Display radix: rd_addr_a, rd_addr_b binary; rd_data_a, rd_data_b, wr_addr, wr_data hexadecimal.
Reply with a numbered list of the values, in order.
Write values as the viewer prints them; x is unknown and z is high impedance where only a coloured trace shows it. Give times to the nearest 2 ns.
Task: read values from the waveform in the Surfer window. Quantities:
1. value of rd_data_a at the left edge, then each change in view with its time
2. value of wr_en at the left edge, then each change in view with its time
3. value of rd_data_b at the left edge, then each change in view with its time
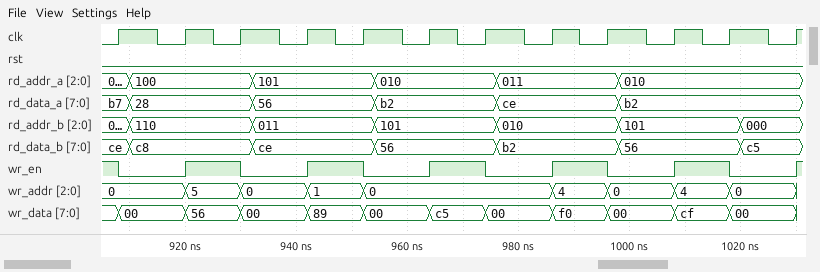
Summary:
1. b7, 28 at 910 ns, 56 at 932 ns, b2 at 954 ns, ce at 976 ns, b2 at 998 ns
2. 1, 0 at 908 ns, 1 at 920 ns, 0 at 930 ns, 1 at 942 ns, 0 at 952 ns, 1 at 964 ns, 0 at 974 ns, 1 at 986 ns, 0 at 996 ns, 1 at 1008 ns, 0 at 1018 ns, 1 at 1030 ns
3. ce, c8 at 910 ns, ce at 932 ns, 56 at 954 ns, b2 at 976 ns, 56 at 998 ns, c5 at 1020 ns
